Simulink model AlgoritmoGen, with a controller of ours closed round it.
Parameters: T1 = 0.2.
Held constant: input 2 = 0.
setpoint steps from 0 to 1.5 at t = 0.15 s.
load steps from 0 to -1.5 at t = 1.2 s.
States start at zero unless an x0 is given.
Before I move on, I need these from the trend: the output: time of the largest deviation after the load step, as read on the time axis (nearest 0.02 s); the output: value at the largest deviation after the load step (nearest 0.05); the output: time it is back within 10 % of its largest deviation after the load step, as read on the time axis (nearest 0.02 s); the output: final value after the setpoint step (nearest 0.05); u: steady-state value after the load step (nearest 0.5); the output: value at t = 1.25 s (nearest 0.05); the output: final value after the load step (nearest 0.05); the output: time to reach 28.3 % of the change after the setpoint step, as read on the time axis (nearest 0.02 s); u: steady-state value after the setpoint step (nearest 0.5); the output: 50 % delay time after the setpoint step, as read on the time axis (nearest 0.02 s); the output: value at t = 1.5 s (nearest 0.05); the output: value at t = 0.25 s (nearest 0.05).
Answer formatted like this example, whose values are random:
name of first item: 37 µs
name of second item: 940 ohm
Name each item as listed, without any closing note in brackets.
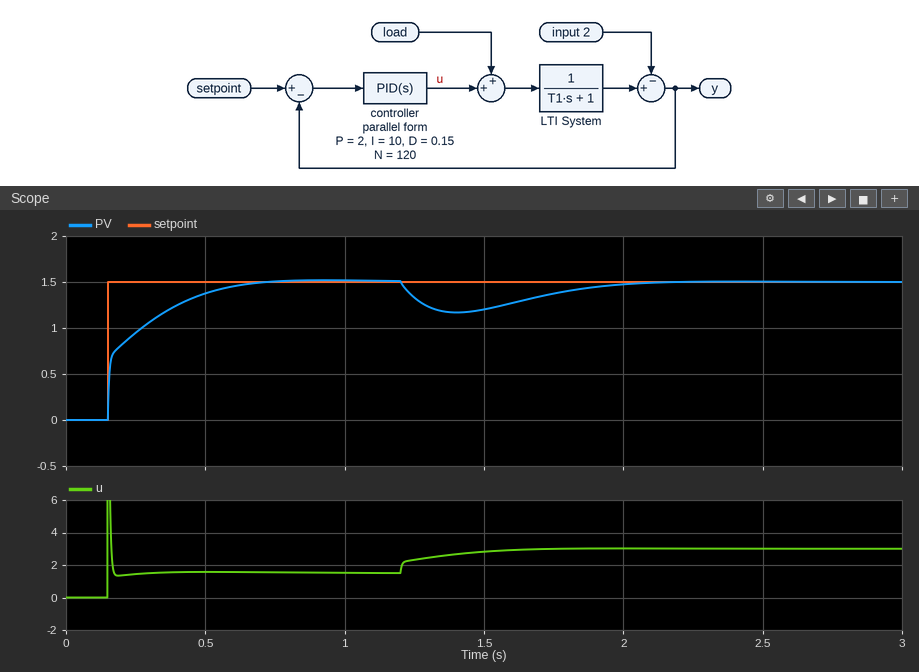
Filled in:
the output: time of the largest deviation after the load step, as read on the time axis: 1.40 s
the output: value at the largest deviation after the load step: 1.15
the output: time it is back within 10 % of its largest deviation after the load step, as read on the time axis: 1.96 s
the output: final value after the setpoint step: 1.50
u: steady-state value after the load step: 3.0
the output: value at t = 1.25 s: 1.35
the output: final value after the load step: 1.50
the output: time to reach 28.3 % of the change after the setpoint step, as read on the time axis: 0.16 s
u: steady-state value after the setpoint step: 1.5
the output: 50 % delay time after the setpoint step, as read on the time axis: 0.18 s
the output: value at t = 1.5 s: 1.20
the output: value at t = 0.25 s: 0.95
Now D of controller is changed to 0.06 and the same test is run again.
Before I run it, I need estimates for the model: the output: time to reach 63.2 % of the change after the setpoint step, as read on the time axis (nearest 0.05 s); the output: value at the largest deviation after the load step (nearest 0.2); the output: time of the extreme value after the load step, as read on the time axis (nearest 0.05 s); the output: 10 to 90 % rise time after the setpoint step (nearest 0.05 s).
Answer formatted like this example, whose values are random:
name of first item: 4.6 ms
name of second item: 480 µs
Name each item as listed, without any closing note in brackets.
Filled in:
the output: time to reach 63.2 % of the change after the setpoint step, as read on the time axis: 0.25 s
the output: value at the largest deviation after the load step: 1.2
the output: time of the extreme value after the load step, as read on the time axis: 1.35 s
the output: 10 to 90 % rise time after the setpoint step: 0.25 s
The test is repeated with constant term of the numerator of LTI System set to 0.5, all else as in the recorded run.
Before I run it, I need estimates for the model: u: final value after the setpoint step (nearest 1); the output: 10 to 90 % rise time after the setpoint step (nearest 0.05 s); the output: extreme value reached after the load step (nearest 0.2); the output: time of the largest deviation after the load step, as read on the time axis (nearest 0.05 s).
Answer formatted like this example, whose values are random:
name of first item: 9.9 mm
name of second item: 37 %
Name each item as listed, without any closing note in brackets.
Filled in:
u: final value after the setpoint step: 3
the output: 10 to 90 % rise time after the setpoint step: 0.55 s
the output: extreme value reached after the load step: 1.2
the output: time of the largest deviation after the load step, as read on the time axis: 1.45 s
